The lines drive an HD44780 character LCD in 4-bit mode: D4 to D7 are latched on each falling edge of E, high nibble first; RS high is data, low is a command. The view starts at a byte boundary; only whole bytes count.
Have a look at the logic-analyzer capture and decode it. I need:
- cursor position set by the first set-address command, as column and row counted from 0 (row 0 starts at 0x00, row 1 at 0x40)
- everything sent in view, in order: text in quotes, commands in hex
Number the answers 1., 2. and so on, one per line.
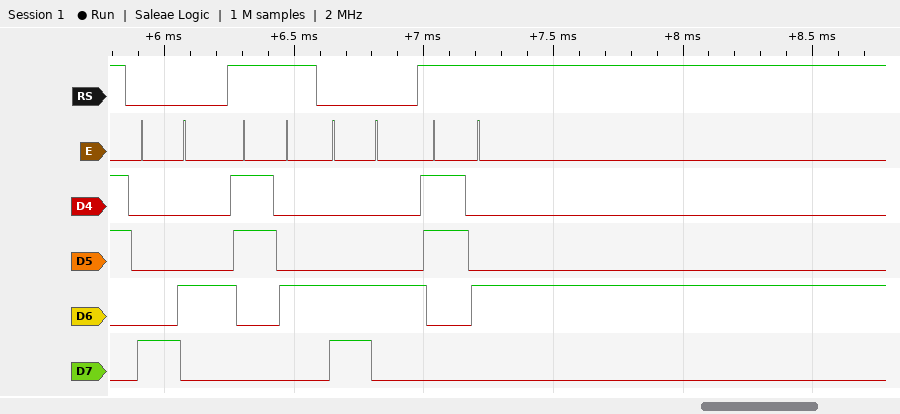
1. column 4, row 0
2. 0x84 "4" 0xC4 "4"
